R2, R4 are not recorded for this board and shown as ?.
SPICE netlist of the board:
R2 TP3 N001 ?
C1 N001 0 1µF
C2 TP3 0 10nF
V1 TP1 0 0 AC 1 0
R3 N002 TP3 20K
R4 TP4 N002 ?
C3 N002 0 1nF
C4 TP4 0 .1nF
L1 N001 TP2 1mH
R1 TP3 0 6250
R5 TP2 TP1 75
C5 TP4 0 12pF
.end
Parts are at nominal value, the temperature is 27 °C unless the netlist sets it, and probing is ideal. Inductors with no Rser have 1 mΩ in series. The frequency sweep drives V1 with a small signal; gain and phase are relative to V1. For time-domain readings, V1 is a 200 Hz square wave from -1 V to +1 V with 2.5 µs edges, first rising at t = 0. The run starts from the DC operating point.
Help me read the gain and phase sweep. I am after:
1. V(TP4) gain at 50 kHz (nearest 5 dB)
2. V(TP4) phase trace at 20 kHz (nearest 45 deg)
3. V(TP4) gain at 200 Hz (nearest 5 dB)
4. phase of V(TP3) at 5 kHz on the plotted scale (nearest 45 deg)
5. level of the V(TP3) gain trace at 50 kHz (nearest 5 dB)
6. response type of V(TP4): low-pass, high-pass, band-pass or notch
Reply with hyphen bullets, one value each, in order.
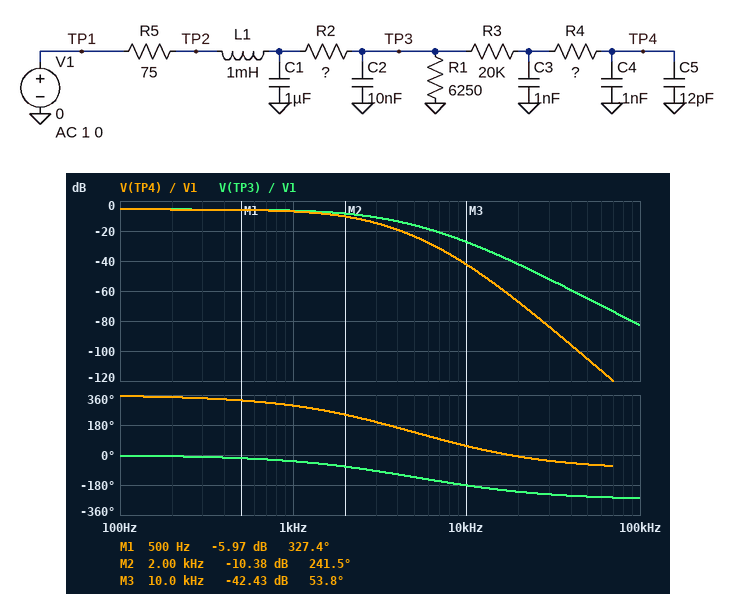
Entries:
- -105 dB
- 0 deg
- -5 dB
- -135 deg
- -65 dB
- low-pass
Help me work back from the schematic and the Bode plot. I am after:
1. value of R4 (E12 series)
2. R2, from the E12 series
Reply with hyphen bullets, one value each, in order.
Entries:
- 470 kΩ
- 5.6 kΩ
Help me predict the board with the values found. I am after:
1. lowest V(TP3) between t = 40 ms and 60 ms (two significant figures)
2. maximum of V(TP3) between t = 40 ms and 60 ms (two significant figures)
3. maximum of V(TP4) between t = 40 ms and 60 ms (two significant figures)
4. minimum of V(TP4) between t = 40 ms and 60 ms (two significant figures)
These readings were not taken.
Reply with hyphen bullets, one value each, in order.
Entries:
- -520 mV
- 520 mV
- 520 mV
- -520 mV
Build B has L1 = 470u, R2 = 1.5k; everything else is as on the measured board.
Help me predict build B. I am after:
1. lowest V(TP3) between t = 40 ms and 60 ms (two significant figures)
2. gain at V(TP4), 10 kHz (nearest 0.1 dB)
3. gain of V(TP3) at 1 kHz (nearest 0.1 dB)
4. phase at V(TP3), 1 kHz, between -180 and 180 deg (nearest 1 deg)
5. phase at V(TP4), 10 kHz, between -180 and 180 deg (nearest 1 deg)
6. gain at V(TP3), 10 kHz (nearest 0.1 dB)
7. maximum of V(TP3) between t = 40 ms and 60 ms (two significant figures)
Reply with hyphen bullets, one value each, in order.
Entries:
- -800 mV
- -32.9 dB
- -2.7 dB
- -30 deg
- 99 deg
- -17.8 dB
- 800 mV
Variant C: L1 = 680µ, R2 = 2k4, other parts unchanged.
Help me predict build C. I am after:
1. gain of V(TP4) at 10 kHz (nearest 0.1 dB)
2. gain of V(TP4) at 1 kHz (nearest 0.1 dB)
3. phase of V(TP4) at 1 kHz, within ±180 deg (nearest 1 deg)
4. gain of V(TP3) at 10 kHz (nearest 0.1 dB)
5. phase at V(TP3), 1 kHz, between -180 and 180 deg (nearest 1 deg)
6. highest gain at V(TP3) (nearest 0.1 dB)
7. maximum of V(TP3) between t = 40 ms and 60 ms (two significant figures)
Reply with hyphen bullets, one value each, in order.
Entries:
- -35.7 dB
- -4.2 dB
- -59 deg
- -20.6 dB
- -33 deg
- -2.9 dB
- 720 mV
